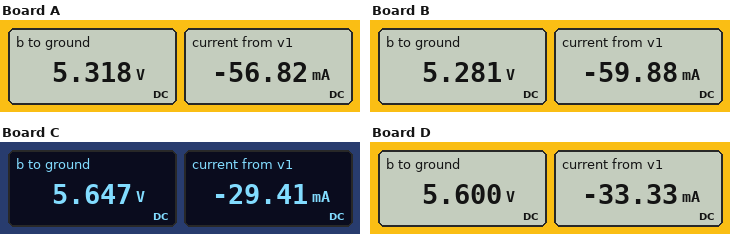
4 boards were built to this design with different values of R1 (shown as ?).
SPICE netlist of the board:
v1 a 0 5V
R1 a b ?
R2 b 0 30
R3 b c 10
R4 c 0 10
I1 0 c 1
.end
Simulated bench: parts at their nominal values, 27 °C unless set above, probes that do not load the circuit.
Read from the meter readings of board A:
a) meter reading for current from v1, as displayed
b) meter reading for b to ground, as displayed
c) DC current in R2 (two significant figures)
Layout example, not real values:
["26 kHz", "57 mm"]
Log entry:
["-56.82 mA", "5.318 V", "180 mA"]
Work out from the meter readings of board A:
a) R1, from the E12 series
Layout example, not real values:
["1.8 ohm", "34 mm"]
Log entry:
["5.6 Ω"]
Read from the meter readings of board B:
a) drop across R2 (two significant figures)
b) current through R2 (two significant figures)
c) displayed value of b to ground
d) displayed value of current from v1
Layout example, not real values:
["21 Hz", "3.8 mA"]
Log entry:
["5.3 V", "180 mA", "5.281 V", "-59.88 mA"]
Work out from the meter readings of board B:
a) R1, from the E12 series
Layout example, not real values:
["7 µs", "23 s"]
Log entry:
["4.7 Ω"]
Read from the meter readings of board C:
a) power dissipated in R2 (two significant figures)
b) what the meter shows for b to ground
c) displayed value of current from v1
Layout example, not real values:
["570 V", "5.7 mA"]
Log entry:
["1.1 W", "5.647 V", "-29.41 mA"]
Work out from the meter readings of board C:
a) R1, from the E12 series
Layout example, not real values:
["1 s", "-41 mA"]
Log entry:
["22 Ω"]
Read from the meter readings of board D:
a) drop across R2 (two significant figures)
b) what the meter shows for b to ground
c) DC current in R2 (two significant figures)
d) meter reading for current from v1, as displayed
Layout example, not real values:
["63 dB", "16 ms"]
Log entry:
["5.6 V", "5.600 V", "190 mA", "-33.33 mA"]
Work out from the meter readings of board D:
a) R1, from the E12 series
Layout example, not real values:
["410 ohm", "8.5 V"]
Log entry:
["18 Ω"]
